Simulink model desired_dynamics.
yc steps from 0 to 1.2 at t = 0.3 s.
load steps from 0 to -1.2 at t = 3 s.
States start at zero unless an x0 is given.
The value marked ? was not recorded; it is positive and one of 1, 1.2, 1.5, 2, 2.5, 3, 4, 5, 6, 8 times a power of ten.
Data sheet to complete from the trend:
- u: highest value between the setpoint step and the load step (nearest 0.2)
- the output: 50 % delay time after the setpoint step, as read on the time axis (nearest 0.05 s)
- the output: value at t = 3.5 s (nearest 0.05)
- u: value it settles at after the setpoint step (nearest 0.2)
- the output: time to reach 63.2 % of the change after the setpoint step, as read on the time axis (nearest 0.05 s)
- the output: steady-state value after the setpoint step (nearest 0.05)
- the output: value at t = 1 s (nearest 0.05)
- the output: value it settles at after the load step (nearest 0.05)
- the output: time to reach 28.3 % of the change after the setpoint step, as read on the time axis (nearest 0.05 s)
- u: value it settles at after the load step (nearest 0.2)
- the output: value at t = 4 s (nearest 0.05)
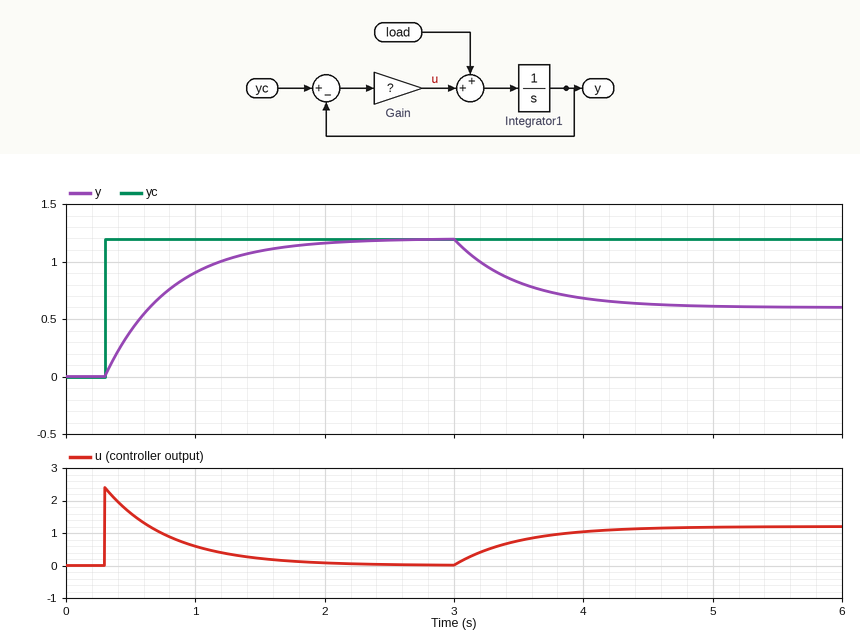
2.4
0.65 s
0.80
0.0
0.80 s
1.20
0.90
0.60
0.45 s
1.2
0.70
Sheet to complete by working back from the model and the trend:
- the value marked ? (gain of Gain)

2
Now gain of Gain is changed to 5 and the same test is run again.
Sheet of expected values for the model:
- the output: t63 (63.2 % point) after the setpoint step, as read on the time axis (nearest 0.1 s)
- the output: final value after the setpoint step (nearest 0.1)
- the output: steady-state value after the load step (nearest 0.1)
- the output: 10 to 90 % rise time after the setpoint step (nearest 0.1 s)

0.5 s
1.2
1.0
0.4 s
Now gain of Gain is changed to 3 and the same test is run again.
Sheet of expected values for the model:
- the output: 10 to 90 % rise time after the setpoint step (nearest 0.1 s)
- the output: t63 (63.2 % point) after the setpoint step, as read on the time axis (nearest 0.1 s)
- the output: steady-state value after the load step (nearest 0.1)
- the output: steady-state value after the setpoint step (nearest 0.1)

0.7 s
0.6 s
0.8
1.2
